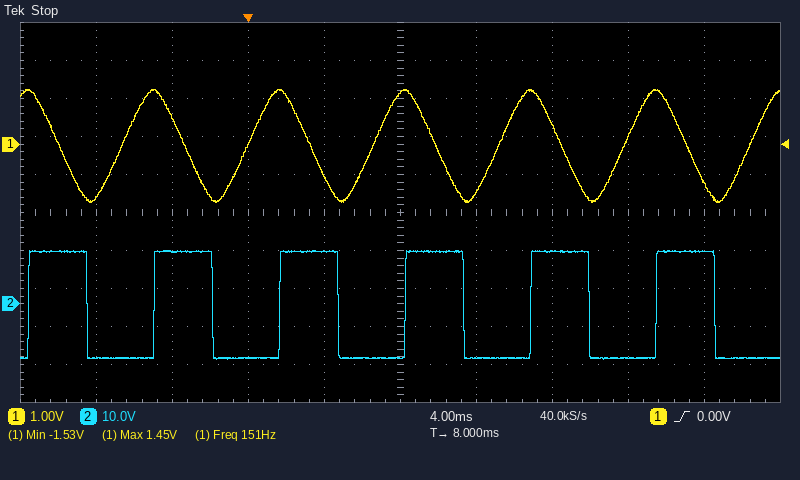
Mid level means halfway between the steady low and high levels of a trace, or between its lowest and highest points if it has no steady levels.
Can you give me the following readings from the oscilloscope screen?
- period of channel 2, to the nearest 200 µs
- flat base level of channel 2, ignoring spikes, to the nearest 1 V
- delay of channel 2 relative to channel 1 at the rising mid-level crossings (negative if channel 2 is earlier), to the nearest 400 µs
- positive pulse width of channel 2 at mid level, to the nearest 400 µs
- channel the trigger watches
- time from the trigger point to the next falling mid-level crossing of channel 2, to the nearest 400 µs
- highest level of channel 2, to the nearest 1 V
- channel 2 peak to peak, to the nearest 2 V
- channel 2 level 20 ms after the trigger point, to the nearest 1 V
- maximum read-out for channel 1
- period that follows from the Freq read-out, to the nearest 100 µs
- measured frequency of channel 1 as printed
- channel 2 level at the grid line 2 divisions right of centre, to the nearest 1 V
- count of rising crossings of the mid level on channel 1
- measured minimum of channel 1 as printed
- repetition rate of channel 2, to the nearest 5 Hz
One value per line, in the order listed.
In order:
6.6 ms
-14 V
+1.6 ms
3.2 ms
channel 1
4.8 ms
14 V
28 V
-14 V
1.45 V
6.6 ms
151 Hz
14 V
6
-1.53 V
150 Hz
